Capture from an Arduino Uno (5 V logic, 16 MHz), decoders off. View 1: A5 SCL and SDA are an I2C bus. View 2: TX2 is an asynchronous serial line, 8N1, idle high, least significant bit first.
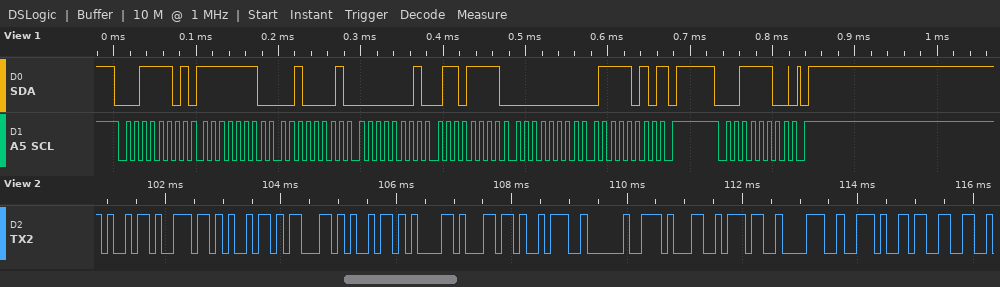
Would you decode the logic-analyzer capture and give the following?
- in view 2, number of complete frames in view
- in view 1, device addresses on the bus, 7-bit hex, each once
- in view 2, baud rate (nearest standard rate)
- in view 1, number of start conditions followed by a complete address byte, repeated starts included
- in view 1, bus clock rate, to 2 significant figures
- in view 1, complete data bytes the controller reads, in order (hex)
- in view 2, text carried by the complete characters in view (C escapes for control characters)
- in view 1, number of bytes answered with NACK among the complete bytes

14
0x1E
9600 baud
2
100 kHz
FE 21 01 6F 00 7A
"inicial: 178.3"
1
